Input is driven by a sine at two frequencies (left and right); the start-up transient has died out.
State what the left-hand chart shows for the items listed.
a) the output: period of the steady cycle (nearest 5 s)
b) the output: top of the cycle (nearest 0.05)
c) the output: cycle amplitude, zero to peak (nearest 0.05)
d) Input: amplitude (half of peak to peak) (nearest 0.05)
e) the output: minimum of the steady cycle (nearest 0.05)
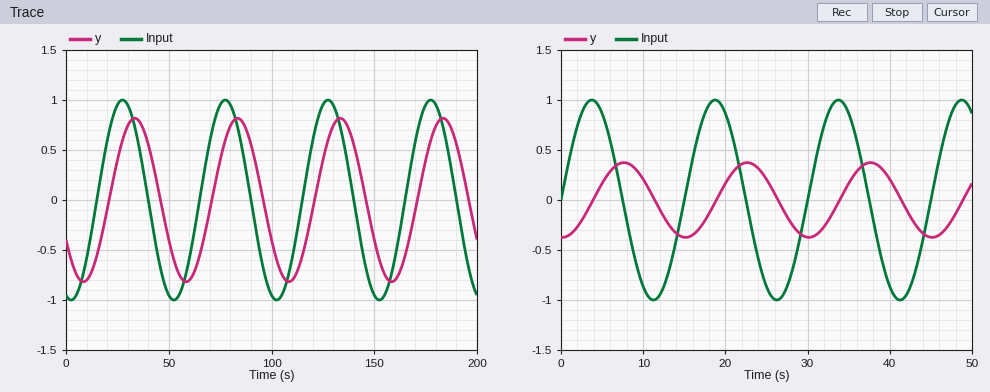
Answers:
50 s
0.80
0.80
1.00
-0.80
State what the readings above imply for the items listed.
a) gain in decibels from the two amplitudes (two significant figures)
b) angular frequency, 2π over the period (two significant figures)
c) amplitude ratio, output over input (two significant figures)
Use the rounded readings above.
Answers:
-1.9 dB
0.13 rad/s
0.80
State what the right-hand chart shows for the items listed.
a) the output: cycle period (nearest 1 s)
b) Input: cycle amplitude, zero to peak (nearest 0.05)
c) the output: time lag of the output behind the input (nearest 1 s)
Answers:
15 s
1.00
4 s
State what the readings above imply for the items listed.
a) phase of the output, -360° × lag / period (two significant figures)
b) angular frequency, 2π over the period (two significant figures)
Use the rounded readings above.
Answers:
-96°
0.42 rad/s
